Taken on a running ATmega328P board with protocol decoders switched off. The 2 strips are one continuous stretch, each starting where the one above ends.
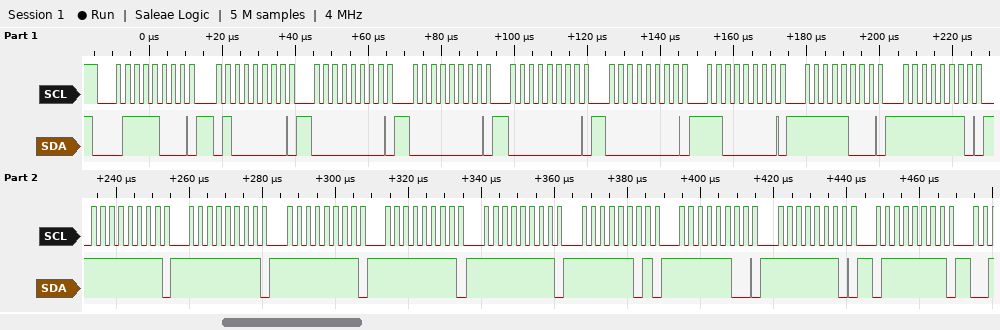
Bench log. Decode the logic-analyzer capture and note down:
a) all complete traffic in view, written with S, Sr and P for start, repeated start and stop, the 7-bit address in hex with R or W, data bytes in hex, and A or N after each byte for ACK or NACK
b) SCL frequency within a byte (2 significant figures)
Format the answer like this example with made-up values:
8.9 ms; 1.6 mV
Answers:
S 3CW A 40 A 00 A 00 A 00 A 00 A C0 A F8 A FE A FF A FF A FF A FF A FF A FD A FC A FE A 7F A; 400 kHz
